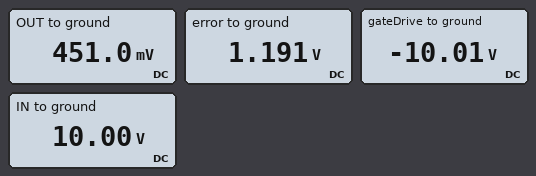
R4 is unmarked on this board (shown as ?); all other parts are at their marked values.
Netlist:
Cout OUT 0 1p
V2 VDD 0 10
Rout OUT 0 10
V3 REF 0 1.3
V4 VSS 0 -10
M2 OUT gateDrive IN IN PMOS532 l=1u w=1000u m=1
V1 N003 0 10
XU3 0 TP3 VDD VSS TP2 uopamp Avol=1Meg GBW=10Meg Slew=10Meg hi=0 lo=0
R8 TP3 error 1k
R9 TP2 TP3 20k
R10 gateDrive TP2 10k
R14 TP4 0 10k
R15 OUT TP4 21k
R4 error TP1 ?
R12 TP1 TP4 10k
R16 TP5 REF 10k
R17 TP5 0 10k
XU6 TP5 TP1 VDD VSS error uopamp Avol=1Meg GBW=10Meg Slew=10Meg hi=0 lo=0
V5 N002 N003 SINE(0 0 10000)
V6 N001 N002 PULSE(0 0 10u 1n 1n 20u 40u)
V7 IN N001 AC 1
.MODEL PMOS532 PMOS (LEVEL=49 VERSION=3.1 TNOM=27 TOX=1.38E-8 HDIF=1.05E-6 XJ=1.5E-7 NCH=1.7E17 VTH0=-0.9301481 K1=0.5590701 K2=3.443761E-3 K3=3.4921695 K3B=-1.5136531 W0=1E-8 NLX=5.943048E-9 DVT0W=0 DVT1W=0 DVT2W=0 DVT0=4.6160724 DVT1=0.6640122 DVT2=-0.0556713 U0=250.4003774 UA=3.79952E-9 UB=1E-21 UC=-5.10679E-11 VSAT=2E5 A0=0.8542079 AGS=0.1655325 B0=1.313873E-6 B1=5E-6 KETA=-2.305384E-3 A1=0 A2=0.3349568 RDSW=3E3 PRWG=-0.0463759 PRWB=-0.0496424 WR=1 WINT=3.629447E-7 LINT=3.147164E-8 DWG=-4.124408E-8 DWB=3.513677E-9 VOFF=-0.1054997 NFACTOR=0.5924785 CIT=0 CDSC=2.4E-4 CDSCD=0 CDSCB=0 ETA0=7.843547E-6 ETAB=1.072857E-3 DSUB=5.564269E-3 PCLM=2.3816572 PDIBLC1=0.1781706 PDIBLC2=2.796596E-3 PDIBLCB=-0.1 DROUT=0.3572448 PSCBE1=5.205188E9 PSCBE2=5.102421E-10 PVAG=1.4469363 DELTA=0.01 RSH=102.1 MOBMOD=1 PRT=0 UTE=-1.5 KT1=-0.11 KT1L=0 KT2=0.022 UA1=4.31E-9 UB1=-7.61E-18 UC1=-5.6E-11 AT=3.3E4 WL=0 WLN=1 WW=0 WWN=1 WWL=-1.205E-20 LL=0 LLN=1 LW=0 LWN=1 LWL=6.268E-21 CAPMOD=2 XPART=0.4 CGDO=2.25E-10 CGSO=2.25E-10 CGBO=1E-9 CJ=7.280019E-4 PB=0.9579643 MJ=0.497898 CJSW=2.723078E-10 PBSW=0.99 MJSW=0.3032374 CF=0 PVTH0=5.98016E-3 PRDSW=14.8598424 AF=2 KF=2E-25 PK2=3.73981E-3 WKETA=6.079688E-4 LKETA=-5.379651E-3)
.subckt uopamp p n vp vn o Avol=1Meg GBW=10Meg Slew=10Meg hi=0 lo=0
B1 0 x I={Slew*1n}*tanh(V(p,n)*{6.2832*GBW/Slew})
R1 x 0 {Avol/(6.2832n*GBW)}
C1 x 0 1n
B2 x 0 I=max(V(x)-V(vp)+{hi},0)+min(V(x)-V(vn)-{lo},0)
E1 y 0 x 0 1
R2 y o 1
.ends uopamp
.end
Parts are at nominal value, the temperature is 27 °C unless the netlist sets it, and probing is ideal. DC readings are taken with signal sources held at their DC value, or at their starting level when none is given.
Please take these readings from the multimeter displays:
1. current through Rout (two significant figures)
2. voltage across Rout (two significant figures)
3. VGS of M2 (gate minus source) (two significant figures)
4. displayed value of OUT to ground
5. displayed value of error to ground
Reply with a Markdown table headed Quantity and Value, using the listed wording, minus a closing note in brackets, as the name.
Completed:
| Quantity | Value |
|---|---|
| current through Rout | 45 mA |
| voltage across Rout | 450 mV |
| VGS of M2 (gate minus source) | -20 V |
| displayed value of OUT to ground | 451.0 mV |
| displayed value of error to ground | 1.191 V |
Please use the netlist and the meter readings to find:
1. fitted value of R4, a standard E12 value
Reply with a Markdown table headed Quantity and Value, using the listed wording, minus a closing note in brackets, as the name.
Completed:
| Quantity | Value |
|---|---|
| fitted value of R4, a standard E12 value | 18 kΩ |
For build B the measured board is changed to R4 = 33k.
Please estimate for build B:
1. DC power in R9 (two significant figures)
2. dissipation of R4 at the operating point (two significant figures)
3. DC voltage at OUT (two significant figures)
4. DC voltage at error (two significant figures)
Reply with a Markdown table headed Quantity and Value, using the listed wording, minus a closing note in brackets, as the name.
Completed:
| Quantity | Value |
|---|---|
| DC power in R9 | 6.2 mW |
| dissipation of R4 at the operating point | 30 µW |
| DC voltage at OUT | 450 mV |
| DC voltage at error | 1.6 V |
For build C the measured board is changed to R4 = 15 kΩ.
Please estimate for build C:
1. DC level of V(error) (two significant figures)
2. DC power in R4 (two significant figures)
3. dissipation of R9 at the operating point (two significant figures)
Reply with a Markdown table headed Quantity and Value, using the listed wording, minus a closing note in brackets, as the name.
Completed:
| Quantity | Value |
|---|---|
| DC level of V(error) | 1.1 V |
| DC power in R4 | 14 µW |
| dissipation of R9 at the operating point | 5.6 mW |
